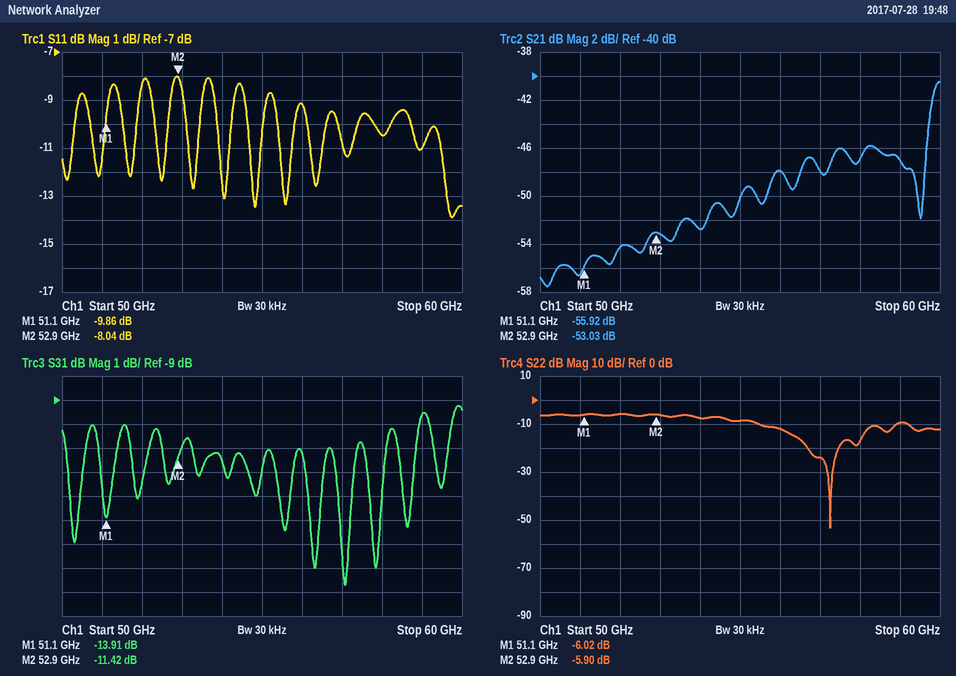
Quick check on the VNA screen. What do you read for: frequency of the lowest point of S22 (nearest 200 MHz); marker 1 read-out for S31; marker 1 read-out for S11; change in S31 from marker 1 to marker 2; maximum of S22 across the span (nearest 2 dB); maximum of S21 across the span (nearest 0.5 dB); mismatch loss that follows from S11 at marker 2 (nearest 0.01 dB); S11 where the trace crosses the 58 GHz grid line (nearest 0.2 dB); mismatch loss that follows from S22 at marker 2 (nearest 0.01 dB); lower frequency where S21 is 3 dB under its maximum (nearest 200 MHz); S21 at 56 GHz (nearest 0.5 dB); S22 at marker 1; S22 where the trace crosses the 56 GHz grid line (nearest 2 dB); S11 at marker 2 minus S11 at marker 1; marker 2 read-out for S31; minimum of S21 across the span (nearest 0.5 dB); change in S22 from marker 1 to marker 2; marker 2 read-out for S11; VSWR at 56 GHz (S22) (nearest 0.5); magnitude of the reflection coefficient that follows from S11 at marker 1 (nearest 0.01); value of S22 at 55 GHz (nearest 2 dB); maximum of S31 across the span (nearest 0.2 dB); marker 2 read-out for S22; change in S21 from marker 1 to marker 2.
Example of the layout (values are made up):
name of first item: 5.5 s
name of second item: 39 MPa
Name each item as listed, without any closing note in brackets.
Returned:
frequency of the lowest point of S22: 57.2 GHz
marker 1 read-out for S31: -13.91 dB
marker 1 read-out for S11: -9.86 dB
change in S31 from marker 1 to marker 2: 2.49 dB
maximum of S22 across the span: -6 dB
maximum of S21 across the span: -40.5 dB
mismatch loss that follows from S11 at marker 2: 0.74 dB
S11 where the trace crosses the 58 GHz grid line: -10.4 dB
mismatch loss that follows from S22 at marker 2: 1.29 dB
lower frequency where S21 is 3 dB under its maximum: 59.8 GHz
S21 at 56 GHz: -48.0 dB
S22 at marker 1: -6.02 dB
S22 where the trace crosses the 56 GHz grid line: -12 dB
S11 at marker 2 minus S11 at marker 1: 1.82 dB
marker 2 read-out for S31: -11.42 dB
minimum of S21 across the span: -57.5 dB
change in S22 from marker 1 to marker 2: 0.12 dB
marker 2 read-out for S11: -8.04 dB
VSWR at 56 GHz (S22): 1.5
magnitude of the reflection coefficient that follows from S11 at marker 1: 0.32
value of S22 at 55 GHz: -8 dB
maximum of S31 across the span: -9.2 dB
marker 2 read-out for S22: -5.90 dB
change in S21 from marker 1 to marker 2: 2.89 dB
